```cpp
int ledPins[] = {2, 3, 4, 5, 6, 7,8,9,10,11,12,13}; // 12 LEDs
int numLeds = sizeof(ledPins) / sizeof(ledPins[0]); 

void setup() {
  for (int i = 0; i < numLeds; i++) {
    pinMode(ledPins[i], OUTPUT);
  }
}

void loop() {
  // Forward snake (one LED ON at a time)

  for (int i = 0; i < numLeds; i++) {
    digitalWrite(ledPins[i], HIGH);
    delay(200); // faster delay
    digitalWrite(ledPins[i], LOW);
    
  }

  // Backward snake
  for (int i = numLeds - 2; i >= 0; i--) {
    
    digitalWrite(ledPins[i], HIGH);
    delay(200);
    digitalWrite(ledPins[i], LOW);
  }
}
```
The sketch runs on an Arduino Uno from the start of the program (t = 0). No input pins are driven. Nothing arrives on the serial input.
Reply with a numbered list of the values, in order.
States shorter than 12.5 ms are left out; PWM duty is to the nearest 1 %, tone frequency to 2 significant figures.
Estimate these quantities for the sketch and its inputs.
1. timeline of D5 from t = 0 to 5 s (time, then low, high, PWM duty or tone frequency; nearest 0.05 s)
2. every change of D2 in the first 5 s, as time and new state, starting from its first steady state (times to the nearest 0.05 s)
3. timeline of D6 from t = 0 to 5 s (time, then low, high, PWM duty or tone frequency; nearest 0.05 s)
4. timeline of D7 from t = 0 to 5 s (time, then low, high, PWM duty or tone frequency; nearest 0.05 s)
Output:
1. 0 s low; 0.6 s high; 0.8 s low; 3.8 s high; 4 s low
2. 0 s high; 0.2 s low; 4.4 s high; 4.8 s low
3. 0 s low; 0.8 s high; 1 s low; 3.6 s high; 3.8 s low
4. 0 s low; 1 s high; 1.2 s low; 3.4 s high; 3.6 s low
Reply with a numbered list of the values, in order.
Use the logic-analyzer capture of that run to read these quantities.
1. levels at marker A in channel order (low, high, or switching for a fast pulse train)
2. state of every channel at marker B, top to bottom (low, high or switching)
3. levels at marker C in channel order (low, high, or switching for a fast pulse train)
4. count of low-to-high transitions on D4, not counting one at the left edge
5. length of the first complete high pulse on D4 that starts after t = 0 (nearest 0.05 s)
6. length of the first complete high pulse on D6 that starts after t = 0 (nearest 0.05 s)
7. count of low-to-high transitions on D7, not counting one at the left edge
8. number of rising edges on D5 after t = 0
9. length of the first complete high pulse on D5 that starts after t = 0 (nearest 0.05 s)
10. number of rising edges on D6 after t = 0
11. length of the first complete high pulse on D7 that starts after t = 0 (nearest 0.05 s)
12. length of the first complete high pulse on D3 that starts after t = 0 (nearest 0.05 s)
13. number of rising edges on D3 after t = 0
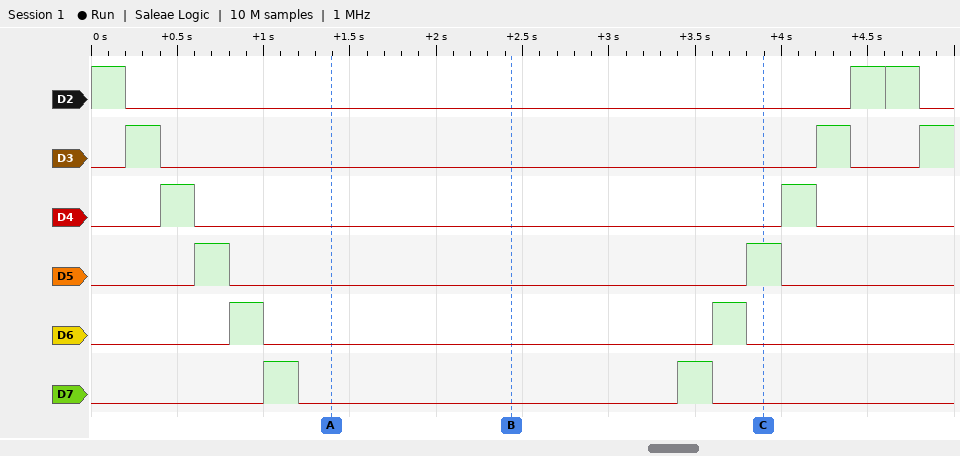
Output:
1. D2 low, D3 low, D4 low, D5 low, D6 low, D7 low
2. D2 low, D3 low, D4 low, D5 low, D6 low, D7 low
3. D2 low, D3 low, D4 low, D5 high, D6 low, D7 low
4. 2
5. 0.20 s
6. 0.20 s
7. 2
8. 2
9. 0.20 s
10. 2
11. 0.20 s
12. 0.20 s
13. 3
